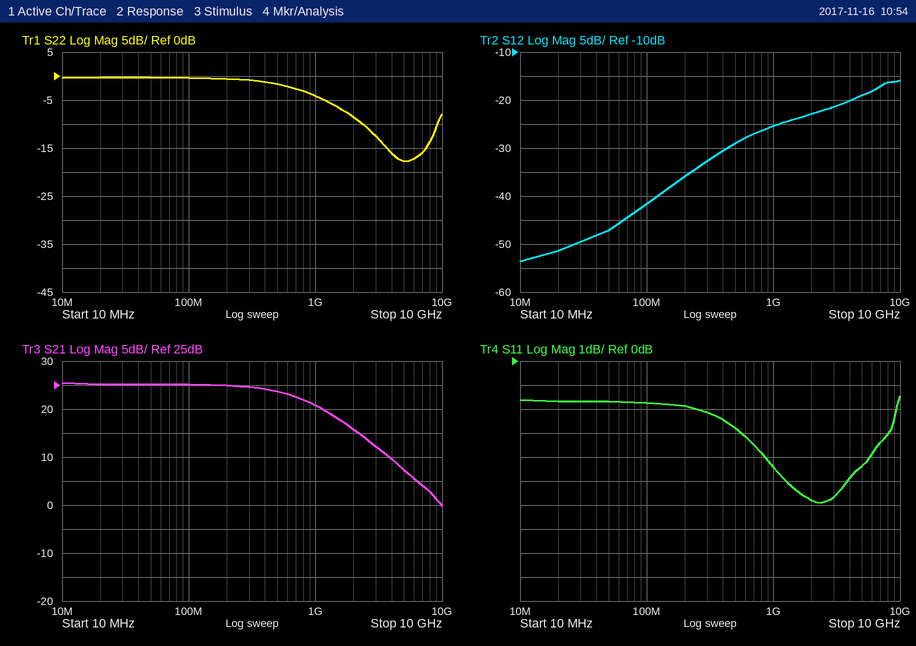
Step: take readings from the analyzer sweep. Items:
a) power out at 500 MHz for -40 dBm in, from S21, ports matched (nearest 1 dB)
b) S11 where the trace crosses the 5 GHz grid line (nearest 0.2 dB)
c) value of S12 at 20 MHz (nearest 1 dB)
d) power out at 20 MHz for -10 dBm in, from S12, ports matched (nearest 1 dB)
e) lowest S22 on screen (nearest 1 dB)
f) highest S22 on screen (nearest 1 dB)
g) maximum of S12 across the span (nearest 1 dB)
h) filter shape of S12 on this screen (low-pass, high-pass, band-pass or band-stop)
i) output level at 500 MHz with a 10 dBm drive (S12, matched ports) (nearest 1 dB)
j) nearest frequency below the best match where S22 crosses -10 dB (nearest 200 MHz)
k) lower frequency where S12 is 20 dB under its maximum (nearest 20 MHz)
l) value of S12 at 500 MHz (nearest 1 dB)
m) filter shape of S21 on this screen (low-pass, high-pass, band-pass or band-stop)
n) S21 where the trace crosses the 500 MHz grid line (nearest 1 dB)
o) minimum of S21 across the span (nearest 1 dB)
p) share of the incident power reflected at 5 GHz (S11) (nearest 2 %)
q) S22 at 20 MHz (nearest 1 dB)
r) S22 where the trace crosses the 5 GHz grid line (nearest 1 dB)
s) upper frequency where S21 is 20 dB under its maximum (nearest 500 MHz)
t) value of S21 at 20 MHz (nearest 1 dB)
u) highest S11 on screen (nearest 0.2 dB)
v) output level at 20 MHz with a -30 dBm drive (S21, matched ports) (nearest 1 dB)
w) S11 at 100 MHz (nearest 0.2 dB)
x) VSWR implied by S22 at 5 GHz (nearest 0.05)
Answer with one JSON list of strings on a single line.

["-16 dBm", "-4.4 dB", "-51 dB", "-61 dBm", "-18 dB", "0 dB", "-16 dB", "high-pass", "-19 dBm", "2.4 GHz", "200 MHz", "-29 dB", "low-pass", "24 dB", "0 dB", "36 %", "0 dB", "-18 dB", "6.0 GHz", "25 dB", "-1.4 dB", "-5 dBm", "-1.8 dB", "1.30"]
